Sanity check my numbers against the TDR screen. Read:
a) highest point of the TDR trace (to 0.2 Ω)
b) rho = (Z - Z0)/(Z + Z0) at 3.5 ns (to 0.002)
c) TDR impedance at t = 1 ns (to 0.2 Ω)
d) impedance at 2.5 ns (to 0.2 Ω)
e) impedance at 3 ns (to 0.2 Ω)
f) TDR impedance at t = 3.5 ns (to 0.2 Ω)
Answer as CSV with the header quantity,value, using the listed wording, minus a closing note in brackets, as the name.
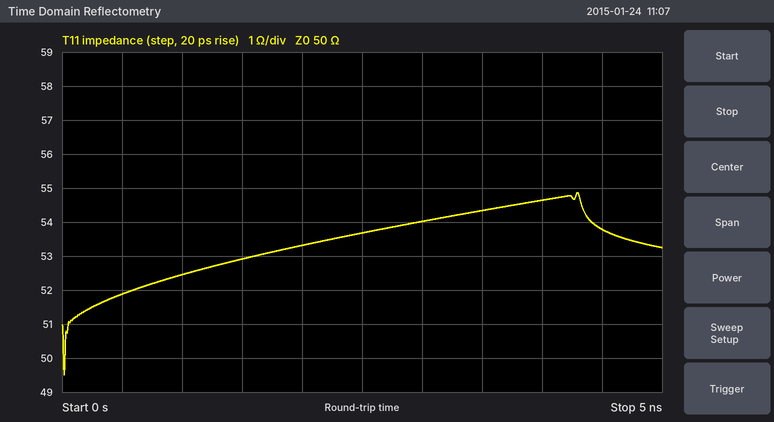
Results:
quantity,value
highest point of the TDR trace,54.8 Ω
rho = (Z - Z0)/(Z + Z0) at 3.5 ns,+0.042
TDR impedance at t = 1 ns,52.4 Ω
impedance at 2.5 ns,53.6 Ω
impedance at 3 ns,54.0 Ω
TDR impedance at t = 3.5 ns,54.4 Ω
